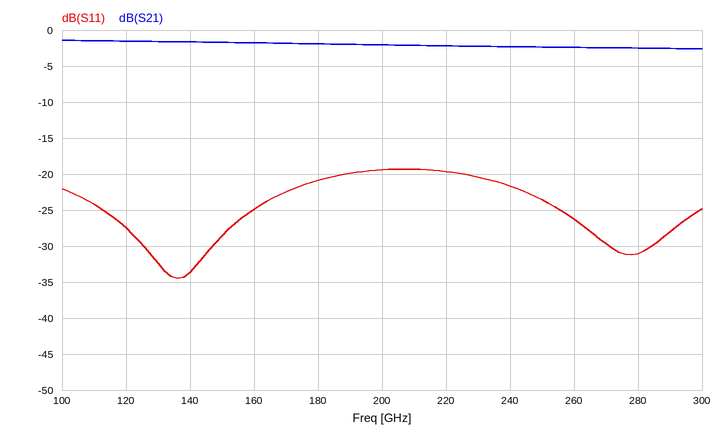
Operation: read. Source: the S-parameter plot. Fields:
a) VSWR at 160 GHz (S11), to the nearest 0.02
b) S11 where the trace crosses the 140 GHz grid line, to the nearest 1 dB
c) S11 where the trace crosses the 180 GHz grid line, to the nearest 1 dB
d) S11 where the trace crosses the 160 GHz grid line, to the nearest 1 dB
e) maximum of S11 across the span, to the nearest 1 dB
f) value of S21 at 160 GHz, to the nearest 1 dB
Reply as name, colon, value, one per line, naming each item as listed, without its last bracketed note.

VSWR at 160 GHz (S11), to the nearest 0.02: 1.12
S11 where the trace crosses the 140 GHz grid line, to the nearest 1 dB: -34 dB
S11 where the trace crosses the 180 GHz grid line, to the nearest 1 dB: -21 dB
S11 where the trace crosses the 160 GHz grid line, to the nearest 1 dB: -25 dB
maximum of S11 across the span, to the nearest 1 dB: -19 dB
value of S21 at 160 GHz, to the nearest 1 dB: -2 dB
